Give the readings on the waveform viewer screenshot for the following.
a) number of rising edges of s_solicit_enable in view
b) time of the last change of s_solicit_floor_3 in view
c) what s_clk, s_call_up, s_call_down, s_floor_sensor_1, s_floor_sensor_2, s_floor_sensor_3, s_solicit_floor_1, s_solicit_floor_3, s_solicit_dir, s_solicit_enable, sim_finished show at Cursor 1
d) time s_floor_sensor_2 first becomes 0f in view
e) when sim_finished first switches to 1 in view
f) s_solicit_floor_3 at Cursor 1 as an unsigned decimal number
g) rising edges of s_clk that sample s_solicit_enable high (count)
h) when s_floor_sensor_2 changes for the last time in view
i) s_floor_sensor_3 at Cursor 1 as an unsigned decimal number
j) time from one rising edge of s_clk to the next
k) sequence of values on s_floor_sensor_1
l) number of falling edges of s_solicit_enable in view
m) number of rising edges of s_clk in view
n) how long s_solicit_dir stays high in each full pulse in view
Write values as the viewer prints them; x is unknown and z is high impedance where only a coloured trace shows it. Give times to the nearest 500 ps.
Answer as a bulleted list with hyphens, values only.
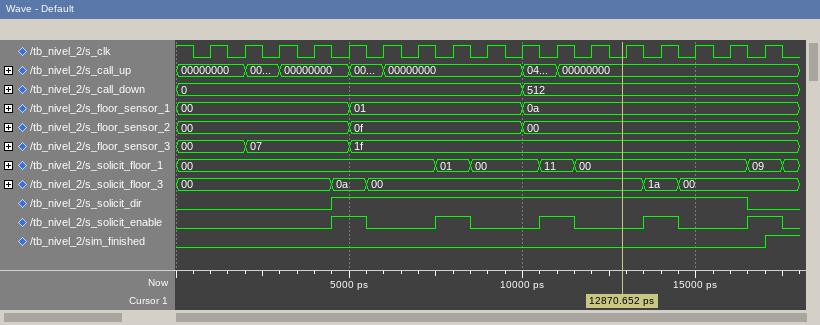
- 5
- 14500 ps
- s_clk=0, s_call_up=00000000, s_call_down=512, s_floor_sensor_1=0a, s_floor_sensor_2=00, s_floor_sensor_3=1f, s_solicit_floor_1=00, s_solicit_floor_3=00, s_solicit_dir=1, s_solicit_enable=0, sim_finished=0
- 5000 ps
- 17000 ps
- 0
- 5
- 10000 ps
- 31
- 1000 ps
- 00, 01, 0a
- 5
- 17
- 12000 ps
